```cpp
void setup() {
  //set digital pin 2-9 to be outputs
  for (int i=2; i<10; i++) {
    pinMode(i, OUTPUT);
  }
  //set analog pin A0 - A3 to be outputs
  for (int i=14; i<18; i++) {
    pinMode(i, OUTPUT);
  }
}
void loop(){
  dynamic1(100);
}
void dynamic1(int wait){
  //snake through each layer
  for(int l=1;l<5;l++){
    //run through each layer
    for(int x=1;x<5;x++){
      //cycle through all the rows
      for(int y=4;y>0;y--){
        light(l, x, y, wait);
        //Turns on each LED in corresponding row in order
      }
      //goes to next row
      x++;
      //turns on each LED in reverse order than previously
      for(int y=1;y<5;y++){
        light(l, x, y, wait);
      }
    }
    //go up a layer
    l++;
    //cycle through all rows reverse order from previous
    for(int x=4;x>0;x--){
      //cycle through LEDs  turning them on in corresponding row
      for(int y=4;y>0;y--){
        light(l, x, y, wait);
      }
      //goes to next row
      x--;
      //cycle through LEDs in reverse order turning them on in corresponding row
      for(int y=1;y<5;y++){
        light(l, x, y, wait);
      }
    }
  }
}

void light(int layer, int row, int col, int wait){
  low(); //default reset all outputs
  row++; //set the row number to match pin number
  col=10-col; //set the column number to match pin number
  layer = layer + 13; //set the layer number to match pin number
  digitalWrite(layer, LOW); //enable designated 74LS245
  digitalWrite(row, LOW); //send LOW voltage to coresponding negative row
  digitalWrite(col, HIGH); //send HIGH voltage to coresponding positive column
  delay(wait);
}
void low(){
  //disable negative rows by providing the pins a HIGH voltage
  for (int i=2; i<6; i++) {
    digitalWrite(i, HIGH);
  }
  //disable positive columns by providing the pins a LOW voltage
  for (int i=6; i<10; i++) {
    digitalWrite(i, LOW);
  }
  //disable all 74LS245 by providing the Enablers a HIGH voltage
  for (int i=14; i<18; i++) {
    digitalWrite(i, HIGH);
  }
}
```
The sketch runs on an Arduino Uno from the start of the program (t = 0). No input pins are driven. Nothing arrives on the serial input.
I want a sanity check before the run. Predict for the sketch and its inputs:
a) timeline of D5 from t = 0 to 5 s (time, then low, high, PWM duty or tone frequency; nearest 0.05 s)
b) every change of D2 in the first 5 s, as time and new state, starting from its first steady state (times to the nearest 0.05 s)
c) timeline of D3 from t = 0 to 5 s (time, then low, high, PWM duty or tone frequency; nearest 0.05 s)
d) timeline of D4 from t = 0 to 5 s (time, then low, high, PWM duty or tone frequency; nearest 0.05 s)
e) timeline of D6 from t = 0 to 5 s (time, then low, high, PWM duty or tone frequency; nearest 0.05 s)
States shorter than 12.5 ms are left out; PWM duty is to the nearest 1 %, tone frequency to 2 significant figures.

0 s high; 1.2 s low; 2 s high; 4.4 s low
0 s low; 0.4 s high; 2.8 s low; 3.6 s high
0 s high; 0.4 s low; 0.8 s high; 2.4 s low; 2.8 s high; 3.6 s low; 4 s high
0 s high; 0.8 s low; 1.2 s high; 2 s low; 2.4 s high; 4 s low; 4.4 s high
0 s high; 0.1 s low; 0.7 s high; 0.9 s low; 1.5 s high; 1.7 s low; 2.3 s high; 2.5 s low; 3.1 s high; 3.3 s low; 3.9 s high; 4.1 s low; 4.7 s high; 4.9 s low
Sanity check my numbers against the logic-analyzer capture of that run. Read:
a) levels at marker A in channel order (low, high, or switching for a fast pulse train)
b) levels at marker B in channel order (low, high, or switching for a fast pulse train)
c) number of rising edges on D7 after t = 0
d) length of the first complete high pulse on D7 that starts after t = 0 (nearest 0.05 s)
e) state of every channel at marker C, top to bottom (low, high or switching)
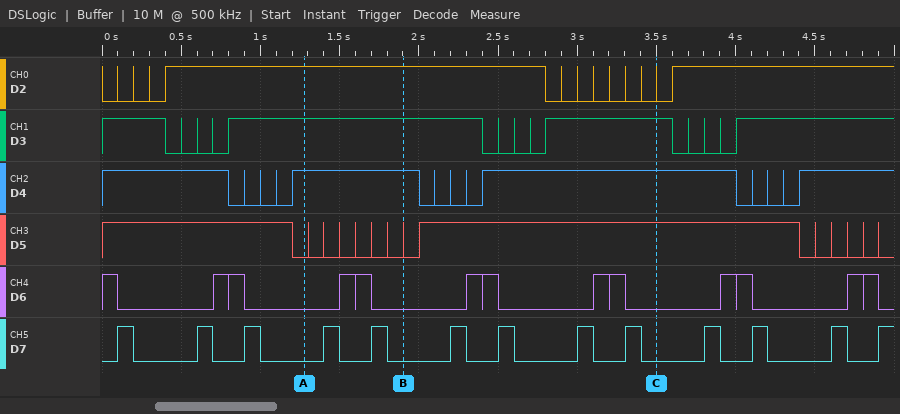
D2 high, D3 high, D4 high, D5 low, D6 low, D7 low
D2 high, D3 high, D4 high, D5 low, D6 low, D7 low
13
0.10 s
D2 low, D3 high, D4 high, D5 high, D6 low, D7 low
